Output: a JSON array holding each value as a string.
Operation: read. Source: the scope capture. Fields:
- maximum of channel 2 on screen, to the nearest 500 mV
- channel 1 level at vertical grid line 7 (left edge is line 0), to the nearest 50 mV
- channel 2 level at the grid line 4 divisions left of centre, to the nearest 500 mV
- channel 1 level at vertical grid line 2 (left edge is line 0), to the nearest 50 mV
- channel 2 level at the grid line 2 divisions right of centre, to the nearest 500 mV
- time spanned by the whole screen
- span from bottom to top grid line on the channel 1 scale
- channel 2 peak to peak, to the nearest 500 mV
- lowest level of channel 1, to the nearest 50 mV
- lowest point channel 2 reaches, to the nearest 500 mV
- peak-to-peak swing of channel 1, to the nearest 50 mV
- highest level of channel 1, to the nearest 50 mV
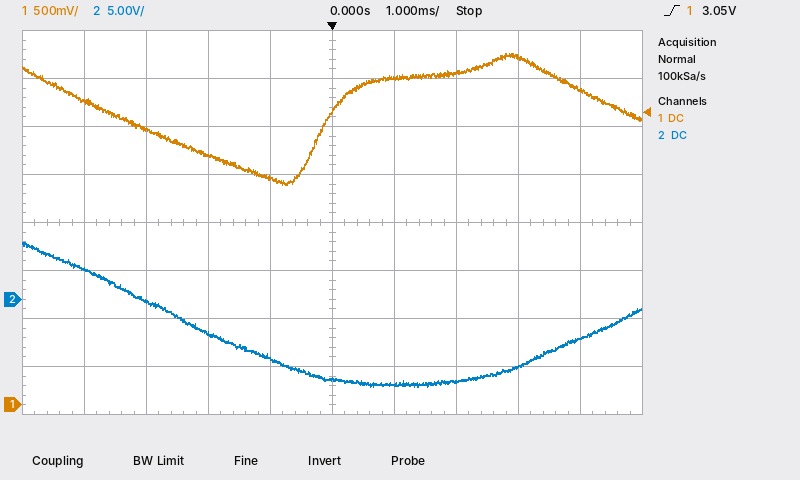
["6.0 V", "3.45 V", "3.0 V", "2.90 V", "-8.5 V", "10 ms", "4 V", "15.0 V", "2.30 V", "-9.0 V", "1.35 V", "3.65 V"]
